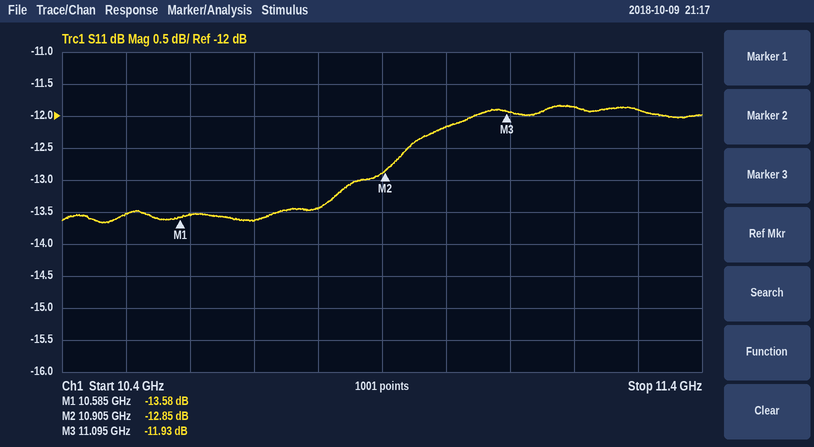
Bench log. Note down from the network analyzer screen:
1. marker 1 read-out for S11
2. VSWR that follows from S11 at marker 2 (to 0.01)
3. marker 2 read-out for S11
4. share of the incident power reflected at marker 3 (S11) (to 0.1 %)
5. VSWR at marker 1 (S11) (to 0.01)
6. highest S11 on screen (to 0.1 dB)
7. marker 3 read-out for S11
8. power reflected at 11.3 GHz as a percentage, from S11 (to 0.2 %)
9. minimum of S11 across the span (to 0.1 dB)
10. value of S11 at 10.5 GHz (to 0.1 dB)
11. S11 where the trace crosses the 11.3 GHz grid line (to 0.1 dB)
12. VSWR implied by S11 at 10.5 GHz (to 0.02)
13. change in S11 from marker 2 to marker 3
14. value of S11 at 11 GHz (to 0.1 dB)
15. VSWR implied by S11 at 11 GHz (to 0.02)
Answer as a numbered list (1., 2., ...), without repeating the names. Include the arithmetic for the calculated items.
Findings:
1. -13.58 dB
2. (1 + 0.2278)/(1 − 0.2278) ≈ 1.59
3. -12.85 dB
4. 10^(-11.93/10) ≈ 6.4 %
5. (1 + 0.2094)/(1 − 0.2094) ≈ 1.53
6. -11.8 dB
7. -11.93 dB
8. 10^(-11.9/10) ≈ 6.46 %, so 6.4 % to the nearest 0.2 %
9. -13.7 dB
10. -13.5 dB
11. -11.9 dB
12. |Γ| = 10^(-13.5/20) = 0.2113; VSWR = (1 + 0.2113)/(1 − 0.2113) ≈ 1.54
13. -11.93 − (-12.85) = 0.92 dB
14. -12.2 dB
15. |Γ| = 10^(-12.2/20) = 0.2455; VSWR = (1 + 0.2455)/(1 − 0.2455) ≈ 1.65, so 1.66 to the nearest 0.02
